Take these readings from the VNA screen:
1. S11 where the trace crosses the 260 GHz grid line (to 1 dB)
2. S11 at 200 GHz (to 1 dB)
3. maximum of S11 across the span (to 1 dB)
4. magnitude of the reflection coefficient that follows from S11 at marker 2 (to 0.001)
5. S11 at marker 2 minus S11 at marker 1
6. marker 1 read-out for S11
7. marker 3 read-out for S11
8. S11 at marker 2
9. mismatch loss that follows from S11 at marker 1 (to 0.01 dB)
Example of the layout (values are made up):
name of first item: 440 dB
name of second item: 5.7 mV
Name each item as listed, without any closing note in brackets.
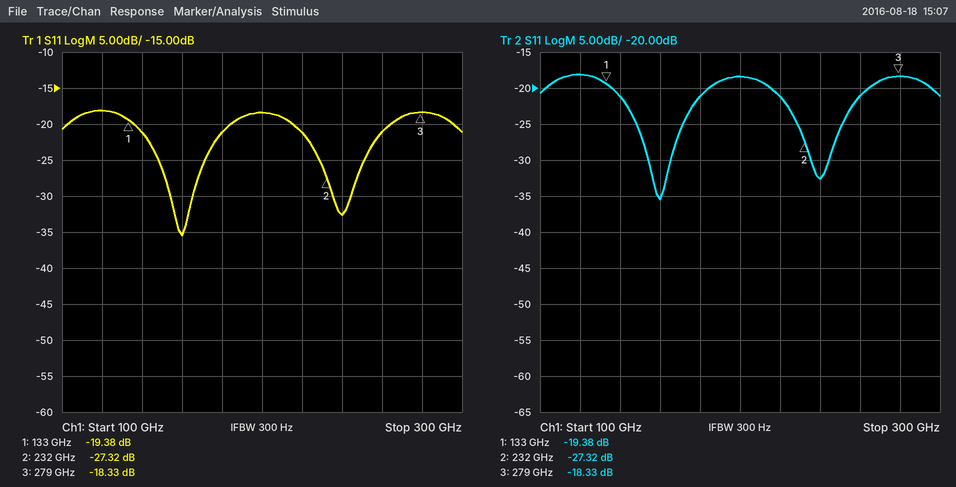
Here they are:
S11 where the trace crosses the 260 GHz grid line: -21 dB
S11 at 200 GHz: -18 dB
maximum of S11 across the span: -18 dB
magnitude of the reflection coefficient that follows from S11 at marker 2: 0.043
S11 at marker 2 minus S11 at marker 1: -7.94 dB
marker 1 read-out for S11: -19.38 dB
marker 3 read-out for S11: -18.33 dB
S11 at marker 2: -27.32 dB
mismatch loss that follows from S11 at marker 1: 0.05 dB
